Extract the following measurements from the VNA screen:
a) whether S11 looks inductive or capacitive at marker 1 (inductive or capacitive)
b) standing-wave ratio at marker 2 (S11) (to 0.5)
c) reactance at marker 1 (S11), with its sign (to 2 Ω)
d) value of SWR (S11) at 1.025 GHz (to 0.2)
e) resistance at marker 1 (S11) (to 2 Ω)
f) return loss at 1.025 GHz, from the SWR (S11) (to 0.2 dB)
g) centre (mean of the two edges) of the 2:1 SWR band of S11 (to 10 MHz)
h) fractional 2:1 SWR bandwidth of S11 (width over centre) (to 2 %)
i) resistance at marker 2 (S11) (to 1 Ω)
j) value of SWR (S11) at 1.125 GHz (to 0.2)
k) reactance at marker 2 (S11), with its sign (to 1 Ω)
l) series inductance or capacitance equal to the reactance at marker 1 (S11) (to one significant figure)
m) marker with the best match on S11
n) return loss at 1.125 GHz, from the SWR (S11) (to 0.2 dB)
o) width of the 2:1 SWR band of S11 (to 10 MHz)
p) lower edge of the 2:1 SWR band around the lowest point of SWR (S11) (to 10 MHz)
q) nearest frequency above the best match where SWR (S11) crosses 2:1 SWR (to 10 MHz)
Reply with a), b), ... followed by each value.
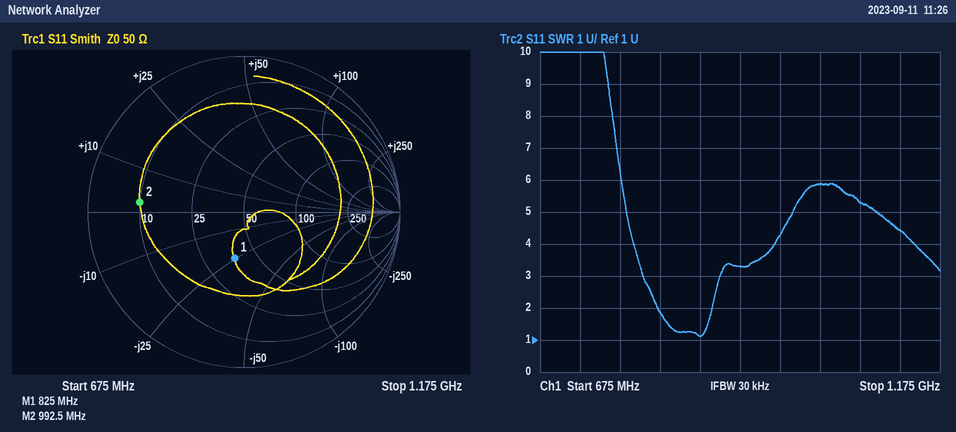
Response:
a) capacitive
b) 5.0
c) -24 Ω
d) 5.8
e) 38 Ω
f) 3.0 dB
g) 860 MHz
h) 8 %
i) 10 Ω
j) 4.4
k) +2 Ω
l) 8 pF
m) marker 1
n) 4.0 dB
o) 70 MHz
p) 820 MHz
q) 890 MHz
